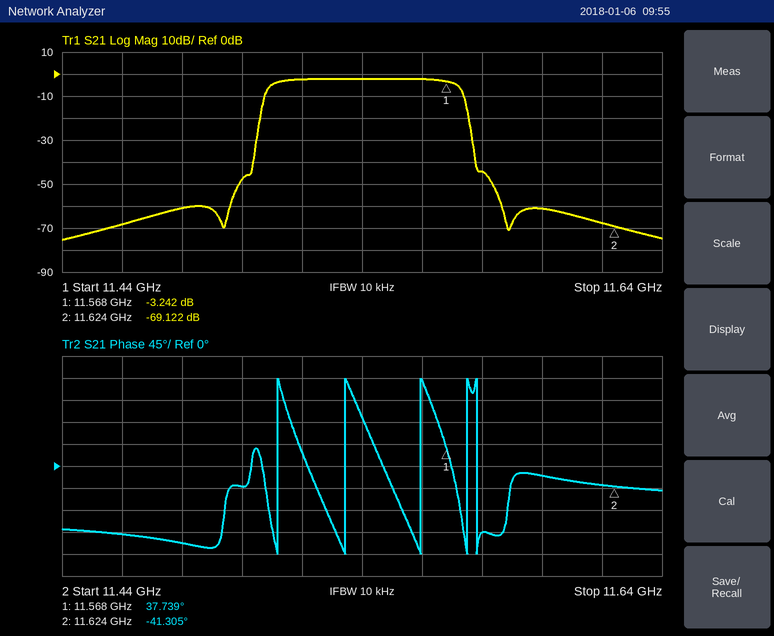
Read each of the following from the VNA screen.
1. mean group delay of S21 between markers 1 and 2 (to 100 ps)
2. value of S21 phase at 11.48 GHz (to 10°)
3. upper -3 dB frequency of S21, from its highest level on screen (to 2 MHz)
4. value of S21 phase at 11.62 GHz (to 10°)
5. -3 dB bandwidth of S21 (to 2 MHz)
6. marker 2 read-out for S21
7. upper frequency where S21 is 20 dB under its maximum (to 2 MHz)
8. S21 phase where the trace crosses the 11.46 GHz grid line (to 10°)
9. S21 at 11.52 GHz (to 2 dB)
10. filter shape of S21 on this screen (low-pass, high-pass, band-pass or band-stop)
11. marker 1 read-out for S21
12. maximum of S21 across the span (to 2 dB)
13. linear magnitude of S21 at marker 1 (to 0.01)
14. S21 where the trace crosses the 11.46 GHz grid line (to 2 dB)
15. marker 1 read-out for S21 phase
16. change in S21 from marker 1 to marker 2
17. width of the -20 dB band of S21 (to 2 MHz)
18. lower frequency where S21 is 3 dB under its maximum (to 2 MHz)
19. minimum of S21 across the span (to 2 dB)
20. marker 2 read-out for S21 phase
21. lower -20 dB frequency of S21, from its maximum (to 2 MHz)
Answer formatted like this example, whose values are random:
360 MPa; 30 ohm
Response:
3.9 ns; -160°; 11.572 GHz; -40°; 62 MHz; -69.122 dB; 11.576 GHz; -140°; -2 dB; band-pass; -3.242 dB; -2 dB; 0.69; -68 dB; 37.739°; -65.880 dB; 70 MHz; 11.510 GHz; -76 dB; -41.305°; 11.506 GHz
